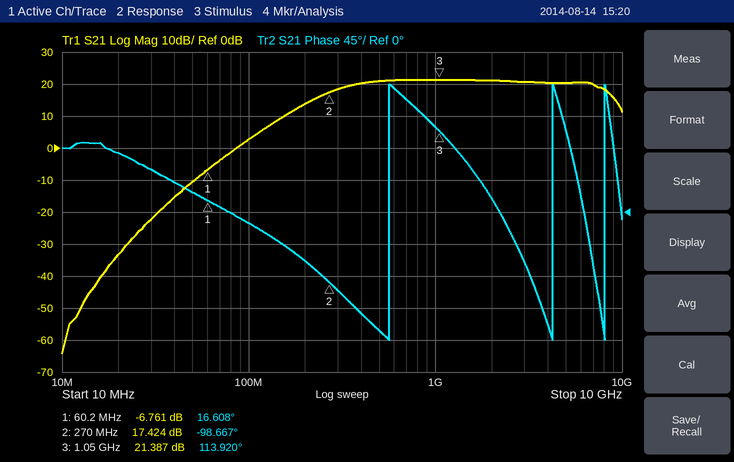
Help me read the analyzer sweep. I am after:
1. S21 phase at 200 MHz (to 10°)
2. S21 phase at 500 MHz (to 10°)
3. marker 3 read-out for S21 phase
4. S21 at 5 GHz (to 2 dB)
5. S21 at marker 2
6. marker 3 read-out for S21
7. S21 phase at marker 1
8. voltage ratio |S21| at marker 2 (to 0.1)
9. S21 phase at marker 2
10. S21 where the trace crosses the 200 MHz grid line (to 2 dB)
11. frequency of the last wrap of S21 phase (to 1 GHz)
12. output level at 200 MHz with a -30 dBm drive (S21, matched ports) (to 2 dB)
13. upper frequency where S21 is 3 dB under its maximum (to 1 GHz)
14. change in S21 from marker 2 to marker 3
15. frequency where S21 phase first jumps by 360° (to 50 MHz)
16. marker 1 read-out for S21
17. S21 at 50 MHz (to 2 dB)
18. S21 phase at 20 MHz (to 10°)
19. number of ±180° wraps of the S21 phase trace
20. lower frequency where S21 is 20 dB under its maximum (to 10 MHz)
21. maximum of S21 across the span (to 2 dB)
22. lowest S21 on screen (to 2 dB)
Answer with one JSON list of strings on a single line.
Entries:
["-70°", "-170°", "113.920°", "20 dB", "17.424 dB", "21.387 dB", "16.608°", "7.4", "-98.667°", "14 dB", "8 GHz", "-16 dBm", "8 GHz", "3.963 dB", "550 MHz", "-6.761 dB", "-10 dB", "80°", "3", "90 MHz", "22 dB", "-64 dB"]
